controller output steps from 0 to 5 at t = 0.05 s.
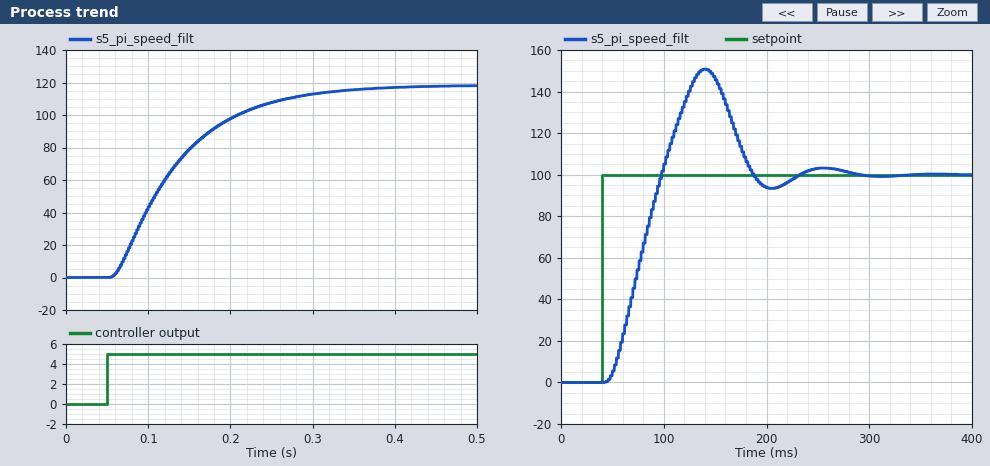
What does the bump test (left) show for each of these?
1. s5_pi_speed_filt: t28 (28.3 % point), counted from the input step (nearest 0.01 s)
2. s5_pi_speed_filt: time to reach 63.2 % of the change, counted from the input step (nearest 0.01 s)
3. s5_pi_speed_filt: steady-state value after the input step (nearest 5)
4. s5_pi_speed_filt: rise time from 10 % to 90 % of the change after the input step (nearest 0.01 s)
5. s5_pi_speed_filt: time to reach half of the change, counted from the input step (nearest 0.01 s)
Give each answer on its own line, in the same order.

0.04 s
0.09 s
120
0.17 s
0.07 s
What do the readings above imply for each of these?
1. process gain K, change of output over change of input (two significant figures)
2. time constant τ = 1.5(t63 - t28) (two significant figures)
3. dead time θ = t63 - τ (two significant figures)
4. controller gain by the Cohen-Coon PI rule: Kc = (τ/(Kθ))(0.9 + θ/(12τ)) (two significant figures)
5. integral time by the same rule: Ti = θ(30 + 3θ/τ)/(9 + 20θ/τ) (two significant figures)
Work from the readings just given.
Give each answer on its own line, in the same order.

24
0.075 s
0.015 s
0.19
0.035 s
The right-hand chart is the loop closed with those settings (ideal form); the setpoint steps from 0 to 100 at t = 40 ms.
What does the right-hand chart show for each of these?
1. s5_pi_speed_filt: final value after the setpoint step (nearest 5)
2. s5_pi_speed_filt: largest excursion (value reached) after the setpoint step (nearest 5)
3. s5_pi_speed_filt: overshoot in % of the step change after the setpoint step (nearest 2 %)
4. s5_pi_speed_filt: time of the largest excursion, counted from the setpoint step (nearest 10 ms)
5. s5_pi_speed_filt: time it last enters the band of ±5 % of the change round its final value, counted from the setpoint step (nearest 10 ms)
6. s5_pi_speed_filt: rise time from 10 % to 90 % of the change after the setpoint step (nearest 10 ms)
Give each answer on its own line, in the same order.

100
150
50 %
100 ms
180 ms
40 ms
